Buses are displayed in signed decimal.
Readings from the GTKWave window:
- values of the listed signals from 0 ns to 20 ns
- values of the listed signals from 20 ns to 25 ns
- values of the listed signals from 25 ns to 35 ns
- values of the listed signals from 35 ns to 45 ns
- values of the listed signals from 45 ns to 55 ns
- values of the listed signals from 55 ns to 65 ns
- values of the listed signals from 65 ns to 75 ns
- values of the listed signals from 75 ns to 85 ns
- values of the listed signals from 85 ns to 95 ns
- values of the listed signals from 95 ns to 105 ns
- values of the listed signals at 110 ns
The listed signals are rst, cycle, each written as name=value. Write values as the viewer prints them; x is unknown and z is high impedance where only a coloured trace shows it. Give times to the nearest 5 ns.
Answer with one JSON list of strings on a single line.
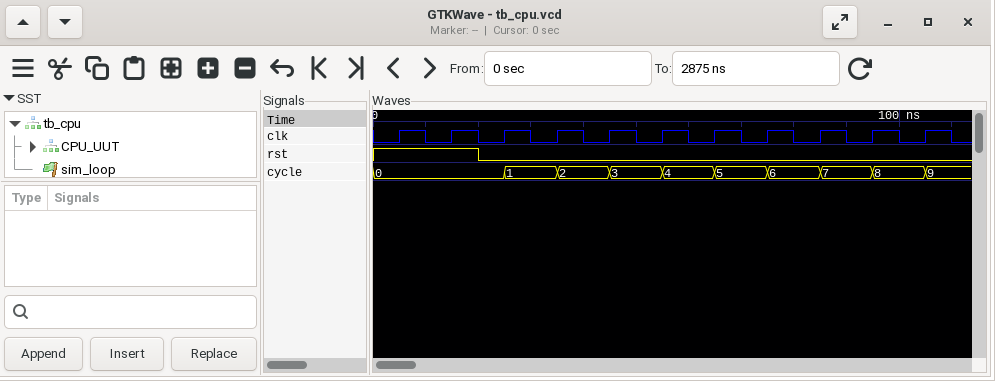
["rst=1, cycle=0", "rst=0, cycle=0", "rst=0, cycle=1", "rst=0, cycle=2", "rst=0, cycle=3", "rst=0, cycle=4", "rst=0, cycle=5", "rst=0, cycle=6", "rst=0, cycle=7", "rst=0, cycle=8", "rst=0, cycle=9"]
